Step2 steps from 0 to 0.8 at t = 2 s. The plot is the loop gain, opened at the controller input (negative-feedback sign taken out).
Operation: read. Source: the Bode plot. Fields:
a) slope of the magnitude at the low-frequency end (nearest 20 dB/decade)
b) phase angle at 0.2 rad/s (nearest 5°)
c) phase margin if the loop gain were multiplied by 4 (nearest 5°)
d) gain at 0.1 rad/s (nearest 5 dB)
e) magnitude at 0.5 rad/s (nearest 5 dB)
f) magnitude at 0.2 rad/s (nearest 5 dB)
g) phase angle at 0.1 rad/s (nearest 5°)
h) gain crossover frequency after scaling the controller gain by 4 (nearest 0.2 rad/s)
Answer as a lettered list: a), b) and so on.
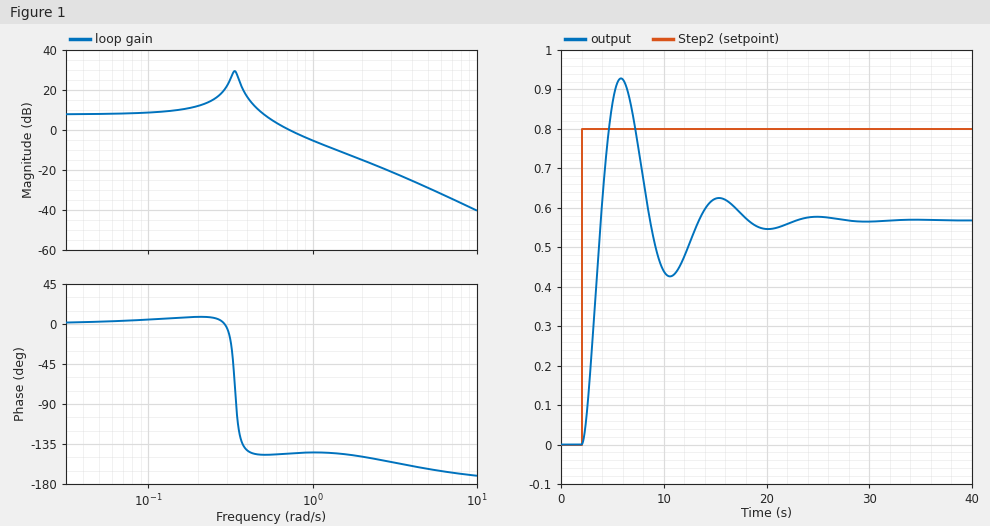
a) 0 dB/decade
b) 10°
c) 35°
d) 10 dB
e) 10 dB
f) 10 dB
g) 5°
h) 1.6 rad/s
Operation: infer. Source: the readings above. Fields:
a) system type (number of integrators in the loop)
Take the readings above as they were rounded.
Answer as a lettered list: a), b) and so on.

a) 0
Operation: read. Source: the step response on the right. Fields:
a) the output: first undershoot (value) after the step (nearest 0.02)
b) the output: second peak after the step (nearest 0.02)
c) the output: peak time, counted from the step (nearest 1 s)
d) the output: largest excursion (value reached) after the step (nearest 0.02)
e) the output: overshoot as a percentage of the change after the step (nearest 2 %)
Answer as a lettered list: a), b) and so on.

a) 0.42
b) 0.62
c) 4 s
d) 0.92
e) 64 %
